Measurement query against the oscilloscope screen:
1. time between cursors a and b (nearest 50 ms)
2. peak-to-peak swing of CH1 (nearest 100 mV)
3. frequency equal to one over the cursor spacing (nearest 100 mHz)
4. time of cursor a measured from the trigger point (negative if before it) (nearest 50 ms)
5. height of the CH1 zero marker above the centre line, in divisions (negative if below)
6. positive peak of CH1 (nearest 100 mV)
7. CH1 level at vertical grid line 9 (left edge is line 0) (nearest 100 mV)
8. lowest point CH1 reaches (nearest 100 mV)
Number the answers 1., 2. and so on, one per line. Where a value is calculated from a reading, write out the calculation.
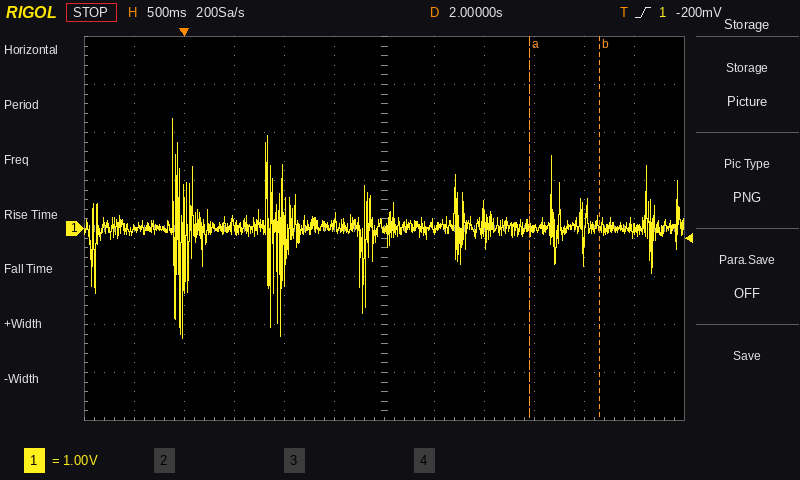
1. 700 ms
2. 2.3 V − (-2.3 V) = 4.6 V
3. 1 / 700 ms ≈ 1.4 Hz
4. +3.45 s
5. 0.0 div
6. 2.3 V
7. 0.0 V
8. -2.3 V
